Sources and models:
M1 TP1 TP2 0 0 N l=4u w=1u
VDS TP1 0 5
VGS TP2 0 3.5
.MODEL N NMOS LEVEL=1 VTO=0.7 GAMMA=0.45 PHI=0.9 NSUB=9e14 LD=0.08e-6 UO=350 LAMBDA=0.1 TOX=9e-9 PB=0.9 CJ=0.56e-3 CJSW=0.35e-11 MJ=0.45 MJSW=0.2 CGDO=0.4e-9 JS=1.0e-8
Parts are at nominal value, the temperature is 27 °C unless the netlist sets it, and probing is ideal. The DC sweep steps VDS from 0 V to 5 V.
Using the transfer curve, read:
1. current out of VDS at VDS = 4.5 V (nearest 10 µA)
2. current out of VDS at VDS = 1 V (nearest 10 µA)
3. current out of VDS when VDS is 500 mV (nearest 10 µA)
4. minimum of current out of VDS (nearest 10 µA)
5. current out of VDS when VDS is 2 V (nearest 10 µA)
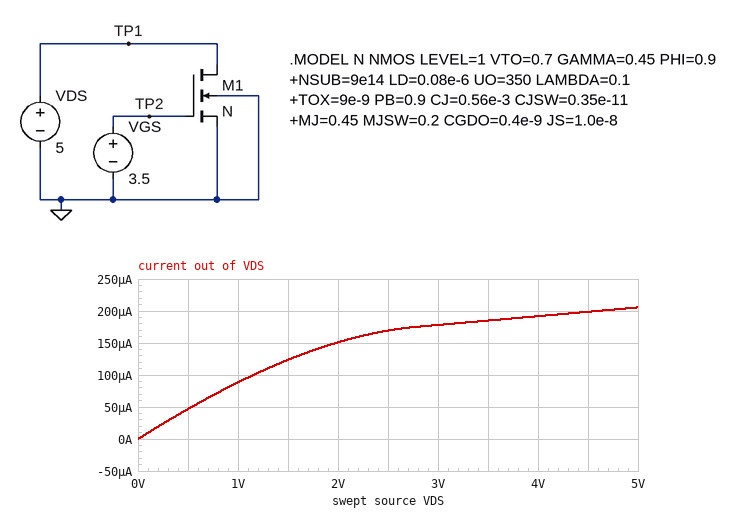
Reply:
200 µA
90 µA
50 µA
0 A
150 µA
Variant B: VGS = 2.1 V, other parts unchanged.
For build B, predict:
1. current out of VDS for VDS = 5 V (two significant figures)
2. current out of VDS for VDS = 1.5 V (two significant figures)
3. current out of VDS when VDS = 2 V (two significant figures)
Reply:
51 µA
39 µA
41 µA
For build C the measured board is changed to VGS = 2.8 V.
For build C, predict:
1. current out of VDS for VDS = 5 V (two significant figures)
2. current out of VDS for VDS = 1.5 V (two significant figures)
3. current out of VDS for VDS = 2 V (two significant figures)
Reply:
120 µA
81 µA
92 µA
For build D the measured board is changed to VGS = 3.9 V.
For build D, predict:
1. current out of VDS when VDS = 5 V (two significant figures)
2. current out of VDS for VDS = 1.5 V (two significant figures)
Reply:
270 µA
150 µA
